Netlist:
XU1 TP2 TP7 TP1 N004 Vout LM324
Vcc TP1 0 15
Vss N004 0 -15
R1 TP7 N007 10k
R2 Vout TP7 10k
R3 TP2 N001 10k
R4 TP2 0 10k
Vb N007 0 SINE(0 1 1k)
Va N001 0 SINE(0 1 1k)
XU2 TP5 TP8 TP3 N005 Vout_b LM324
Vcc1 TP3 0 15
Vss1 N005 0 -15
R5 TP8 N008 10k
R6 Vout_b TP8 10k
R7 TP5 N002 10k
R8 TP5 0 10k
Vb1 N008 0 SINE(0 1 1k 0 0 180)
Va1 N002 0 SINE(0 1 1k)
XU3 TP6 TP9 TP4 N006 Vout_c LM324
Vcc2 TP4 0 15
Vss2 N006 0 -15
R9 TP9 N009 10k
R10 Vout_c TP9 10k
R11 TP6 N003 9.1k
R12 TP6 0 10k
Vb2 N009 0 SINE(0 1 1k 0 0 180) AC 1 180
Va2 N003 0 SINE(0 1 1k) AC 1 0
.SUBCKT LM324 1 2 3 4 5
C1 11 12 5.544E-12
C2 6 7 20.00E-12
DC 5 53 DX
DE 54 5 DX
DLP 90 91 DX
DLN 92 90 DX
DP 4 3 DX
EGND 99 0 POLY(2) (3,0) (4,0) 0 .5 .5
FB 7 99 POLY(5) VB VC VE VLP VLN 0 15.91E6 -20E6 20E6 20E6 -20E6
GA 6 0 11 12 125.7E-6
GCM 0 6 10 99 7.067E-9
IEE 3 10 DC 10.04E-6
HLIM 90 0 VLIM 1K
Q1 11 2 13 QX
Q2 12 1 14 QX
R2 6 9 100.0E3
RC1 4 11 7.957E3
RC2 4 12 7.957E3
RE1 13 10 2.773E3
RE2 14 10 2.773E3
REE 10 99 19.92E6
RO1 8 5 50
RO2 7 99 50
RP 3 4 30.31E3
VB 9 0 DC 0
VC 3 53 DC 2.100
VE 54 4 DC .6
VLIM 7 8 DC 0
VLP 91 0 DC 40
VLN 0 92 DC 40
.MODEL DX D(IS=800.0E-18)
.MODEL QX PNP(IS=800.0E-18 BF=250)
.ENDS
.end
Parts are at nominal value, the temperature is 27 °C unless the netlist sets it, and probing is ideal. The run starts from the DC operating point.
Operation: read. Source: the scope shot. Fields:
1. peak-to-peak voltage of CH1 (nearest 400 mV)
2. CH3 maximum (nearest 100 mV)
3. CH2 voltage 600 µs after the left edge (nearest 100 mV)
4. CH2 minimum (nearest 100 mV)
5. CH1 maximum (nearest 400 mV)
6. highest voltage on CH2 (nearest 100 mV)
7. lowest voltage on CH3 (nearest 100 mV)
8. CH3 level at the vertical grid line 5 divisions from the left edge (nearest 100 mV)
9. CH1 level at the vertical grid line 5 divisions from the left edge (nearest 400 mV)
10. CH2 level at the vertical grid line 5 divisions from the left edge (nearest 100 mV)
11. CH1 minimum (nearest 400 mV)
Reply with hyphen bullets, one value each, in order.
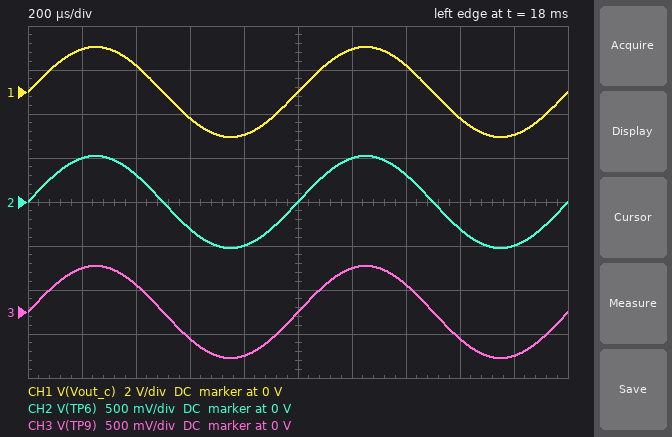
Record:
- 4.0 V
- 500 mV
- -300 mV
- -500 mV
- 2.0 V
- 500 mV
- -500 mV
- 0 V
- 0 V
- 0 V
- -2.0 V
